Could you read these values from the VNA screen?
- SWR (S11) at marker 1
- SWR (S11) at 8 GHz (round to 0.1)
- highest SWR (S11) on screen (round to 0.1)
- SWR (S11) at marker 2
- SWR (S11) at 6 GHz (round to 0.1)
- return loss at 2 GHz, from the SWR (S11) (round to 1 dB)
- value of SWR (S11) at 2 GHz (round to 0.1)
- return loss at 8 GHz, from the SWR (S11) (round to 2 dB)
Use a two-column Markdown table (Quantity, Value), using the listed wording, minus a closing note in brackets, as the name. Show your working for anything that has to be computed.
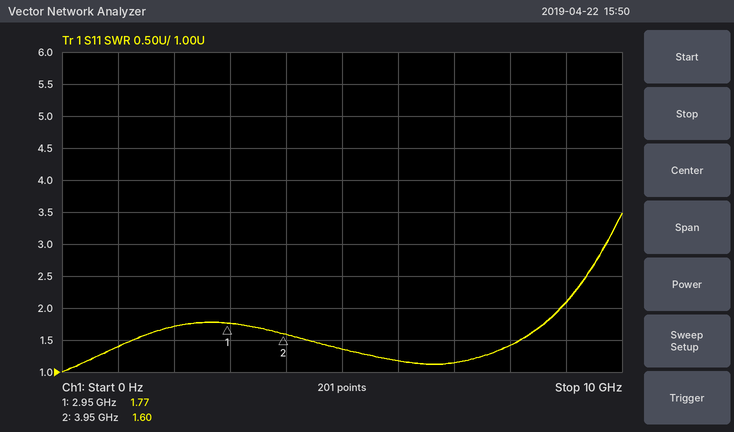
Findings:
| Quantity | Value |
|---|---|
| SWR (S11) at marker 1 | 1.77 |
| SWR (S11) at 8 GHz | 1.4 |
| highest SWR (S11) on screen | 3.5 |
| SWR (S11) at marker 2 | 1.60 |
| SWR (S11) at 6 GHz | 1.2 |
| return loss at 2 GHz, from the SWR (S11) | −20 log10((1.7 − 1)/(1.7 + 1)) ≈ 12 dB |
| value of SWR (S11) at 2 GHz | 1.7 |
| return loss at 8 GHz, from the SWR (S11) | −20 log10((1.4 − 1)/(1.4 + 1)) ≈ 16 dB |
